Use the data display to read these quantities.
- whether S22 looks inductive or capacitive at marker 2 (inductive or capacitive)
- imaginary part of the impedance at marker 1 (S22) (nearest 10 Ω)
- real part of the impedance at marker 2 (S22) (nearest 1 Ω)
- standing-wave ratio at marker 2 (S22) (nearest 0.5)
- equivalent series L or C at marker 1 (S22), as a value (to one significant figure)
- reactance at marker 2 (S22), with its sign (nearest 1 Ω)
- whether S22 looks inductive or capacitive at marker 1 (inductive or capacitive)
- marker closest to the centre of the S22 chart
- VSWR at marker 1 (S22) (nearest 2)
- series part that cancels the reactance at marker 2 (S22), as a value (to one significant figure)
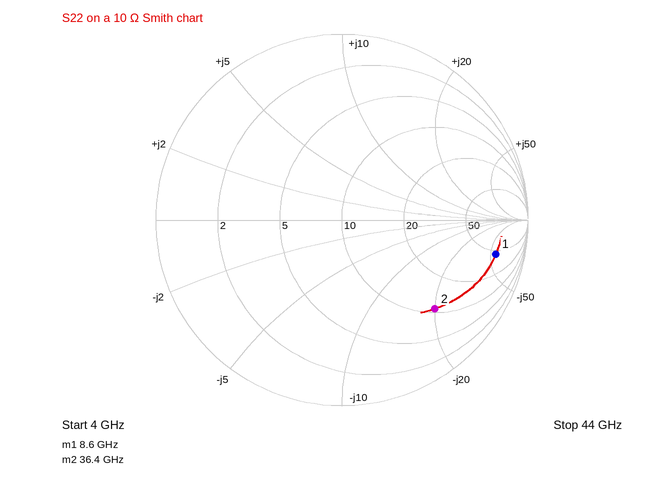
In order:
capacitive
-60 Ω
11 Ω
5.5
300 fF
-20 Ω
capacitive
marker 2
12
90 pH
